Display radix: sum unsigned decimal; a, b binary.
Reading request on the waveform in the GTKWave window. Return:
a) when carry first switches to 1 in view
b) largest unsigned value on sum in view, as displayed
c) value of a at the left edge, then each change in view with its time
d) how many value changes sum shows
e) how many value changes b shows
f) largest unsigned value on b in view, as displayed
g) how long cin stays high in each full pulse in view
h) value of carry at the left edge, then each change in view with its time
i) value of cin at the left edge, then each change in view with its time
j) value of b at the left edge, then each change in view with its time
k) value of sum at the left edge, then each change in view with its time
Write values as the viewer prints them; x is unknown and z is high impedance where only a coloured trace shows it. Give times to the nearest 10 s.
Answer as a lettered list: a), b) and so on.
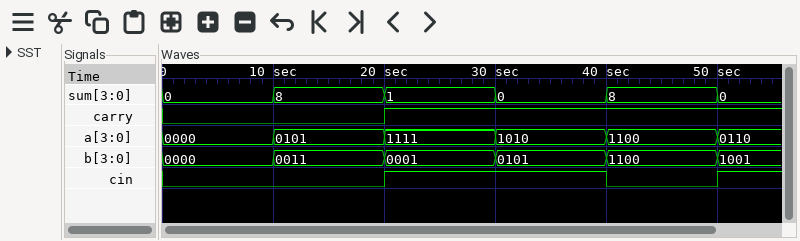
a) 20 s
b) 8
c) 0000, 0101 at 10 s, 1111 at 20 s, 1010 at 30 s, 1100 at 40 s, 0110 at 50 s
d) 5
e) 5
f) 1100
g) 20 s
h) 0, 1 at 20 s
i) 0, 1 at 20 s, 0 at 40 s, 1 at 50 s
j) 0000, 0011 at 10 s, 0001 at 20 s, 0101 at 30 s, 1100 at 40 s, 1001 at 50 s
k) 0, 8 at 10 s, 1 at 20 s, 0 at 30 s, 8 at 40 s, 0 at 50 s
